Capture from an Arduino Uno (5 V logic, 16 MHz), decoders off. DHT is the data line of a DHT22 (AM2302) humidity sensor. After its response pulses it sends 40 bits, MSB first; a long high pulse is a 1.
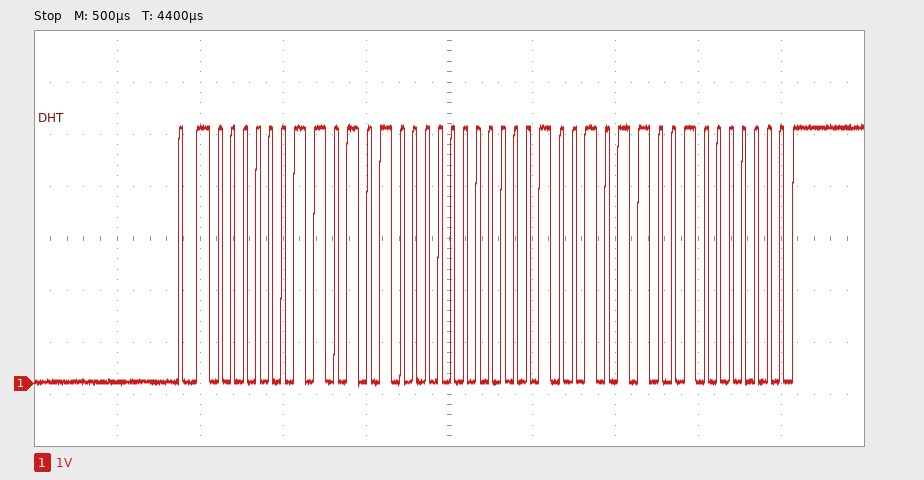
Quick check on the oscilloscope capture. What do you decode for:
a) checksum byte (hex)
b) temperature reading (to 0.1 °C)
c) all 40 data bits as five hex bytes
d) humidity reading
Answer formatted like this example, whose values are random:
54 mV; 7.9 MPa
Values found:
0x80; 30.0 °C; 03 50 01 2C 80; 84.8 %
